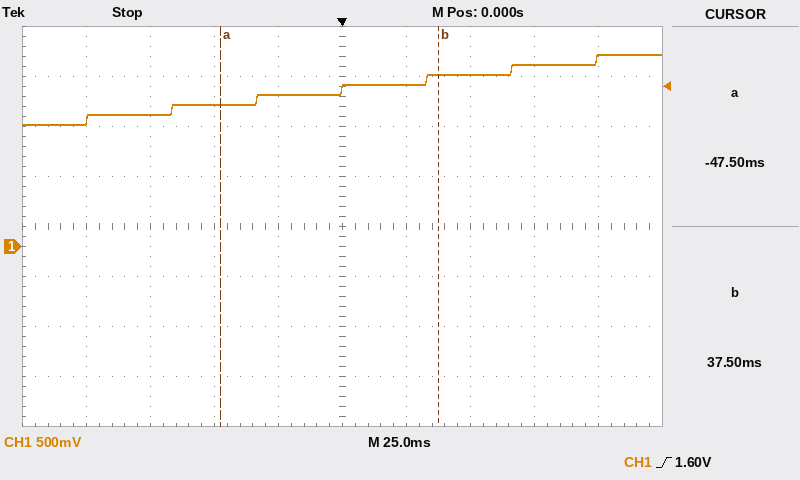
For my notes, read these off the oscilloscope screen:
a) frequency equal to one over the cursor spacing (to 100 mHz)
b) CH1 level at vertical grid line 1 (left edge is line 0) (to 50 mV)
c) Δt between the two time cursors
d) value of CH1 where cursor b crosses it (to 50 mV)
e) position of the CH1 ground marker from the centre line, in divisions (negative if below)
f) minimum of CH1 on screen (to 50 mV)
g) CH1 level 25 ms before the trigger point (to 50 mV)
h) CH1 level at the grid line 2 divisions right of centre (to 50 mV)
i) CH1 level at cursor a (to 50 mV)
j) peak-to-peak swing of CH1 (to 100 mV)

11.8 Hz
1.25 V
85.0 ms
1.70 V
-0.4 div
1.20 V
1.50 V
1.70 V
1.40 V
700 mV
